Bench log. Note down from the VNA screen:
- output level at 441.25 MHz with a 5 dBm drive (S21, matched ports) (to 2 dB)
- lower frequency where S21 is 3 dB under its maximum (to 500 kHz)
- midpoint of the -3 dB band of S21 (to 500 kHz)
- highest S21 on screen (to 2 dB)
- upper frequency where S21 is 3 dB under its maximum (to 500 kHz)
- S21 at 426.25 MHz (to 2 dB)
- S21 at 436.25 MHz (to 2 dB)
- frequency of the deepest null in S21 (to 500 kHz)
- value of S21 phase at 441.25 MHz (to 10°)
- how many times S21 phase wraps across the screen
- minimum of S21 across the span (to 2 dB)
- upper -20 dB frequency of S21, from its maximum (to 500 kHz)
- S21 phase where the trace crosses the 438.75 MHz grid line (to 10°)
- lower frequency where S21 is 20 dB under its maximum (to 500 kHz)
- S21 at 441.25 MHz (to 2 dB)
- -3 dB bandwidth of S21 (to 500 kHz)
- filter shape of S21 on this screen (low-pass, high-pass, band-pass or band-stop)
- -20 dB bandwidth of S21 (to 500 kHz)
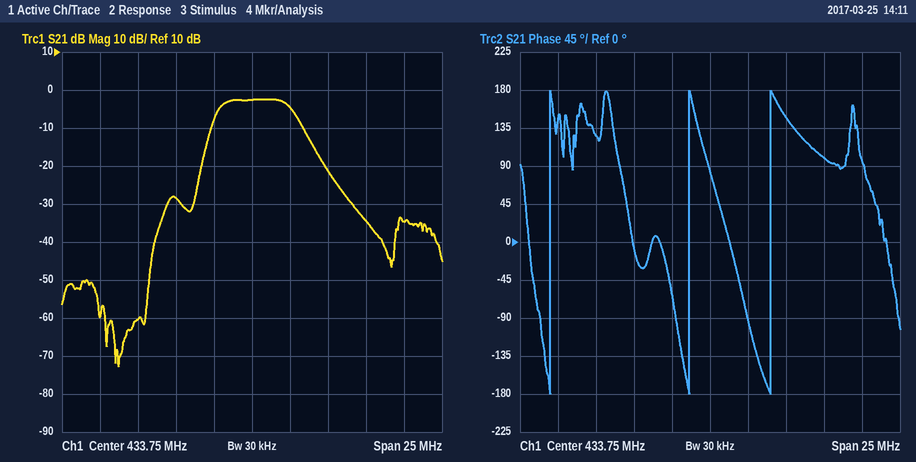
-30 dBm
431.5 MHz
434.0 MHz
-2 dB
436.5 MHz
-60 dB
-4 dB
425.0 MHz
100°
3
-72 dB
439.0 MHz
150°
430.5 MHz
-34 dB
5.0 MHz
band-pass
8.5 MHz
